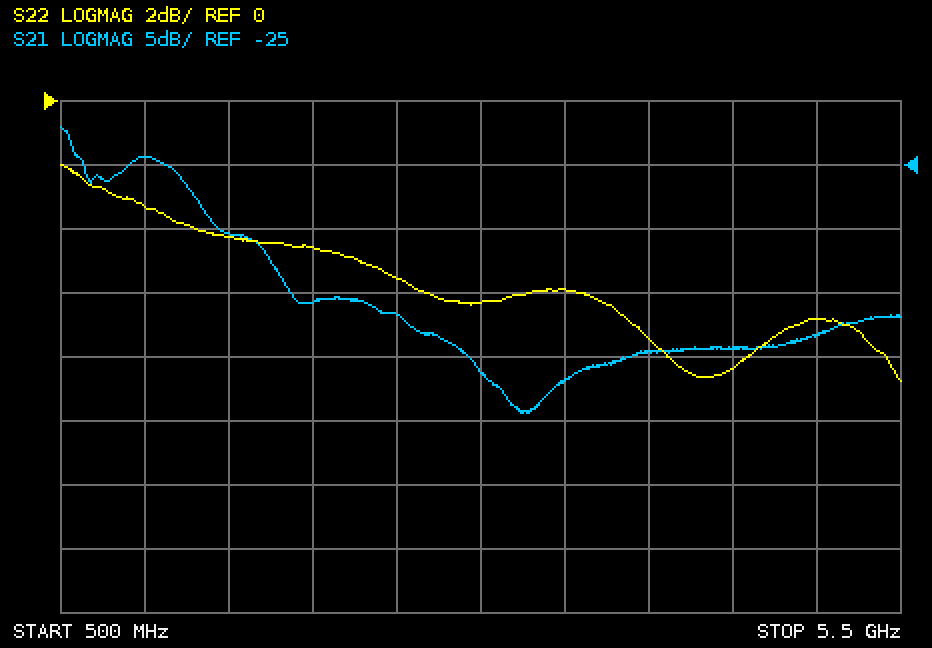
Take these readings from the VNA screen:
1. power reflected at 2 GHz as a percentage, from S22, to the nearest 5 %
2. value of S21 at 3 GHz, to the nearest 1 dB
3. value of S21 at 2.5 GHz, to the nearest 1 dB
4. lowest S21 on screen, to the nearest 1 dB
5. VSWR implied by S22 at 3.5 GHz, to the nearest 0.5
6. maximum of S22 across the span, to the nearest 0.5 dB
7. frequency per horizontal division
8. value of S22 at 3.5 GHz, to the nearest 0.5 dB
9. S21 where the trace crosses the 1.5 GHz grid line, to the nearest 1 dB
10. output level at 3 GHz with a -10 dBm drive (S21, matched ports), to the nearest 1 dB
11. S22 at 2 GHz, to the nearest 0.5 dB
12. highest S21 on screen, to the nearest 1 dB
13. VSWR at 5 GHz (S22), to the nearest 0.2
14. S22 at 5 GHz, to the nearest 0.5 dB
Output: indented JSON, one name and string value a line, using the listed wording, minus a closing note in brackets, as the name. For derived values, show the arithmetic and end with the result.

{
  "power reflected at 2 GHz as a percentage, from S22, to the nearest 5 %": "10^(-4.5/10) ≈ 35 %",
  "value of S21 at 3 GHz, to the nearest 1 dB": "-41 dB",
  "value of S21 at 2.5 GHz, to the nearest 1 dB": "-37 dB",
  "lowest S21 on screen, to the nearest 1 dB": "-44 dB",
  "VSWR implied by S22 at 3.5 GHz, to the nearest 0.5": "|Γ| = 10^(-6/20) = 0.5012; VSWR = (1 + 0.5012)/(1 − 0.5012) ≈ 3.0",
  "maximum of S22 across the span, to the nearest 0.5 dB": "-2.0 dB",
  "frequency per horizontal division": "500 MHz",
  "value of S22 at 3.5 GHz, to the nearest 0.5 dB": "-6.0 dB",
  "S21 where the trace crosses the 1.5 GHz grid line, to the nearest 1 dB": "-30 dB",
  "output level at 3 GHz with a -10 dBm drive (S21, matched ports), to the nearest 1 dB": "-10 dBm + (-41 dB) = -51 dBm",
  "S22 at 2 GHz, to the nearest 0.5 dB": "-4.5 dB",
  "highest S21 on screen, to the nearest 1 dB": "-22 dB",
  "VSWR at 5 GHz (S22), to the nearest 0.2": "|Γ| = 10^(-7/20) = 0.4467; VSWR = (1 + 0.4467)/(1 − 0.4467) ≈ 2.6",
  "S22 at 5 GHz, to the nearest 0.5 dB": "-7.0 dB"
}
